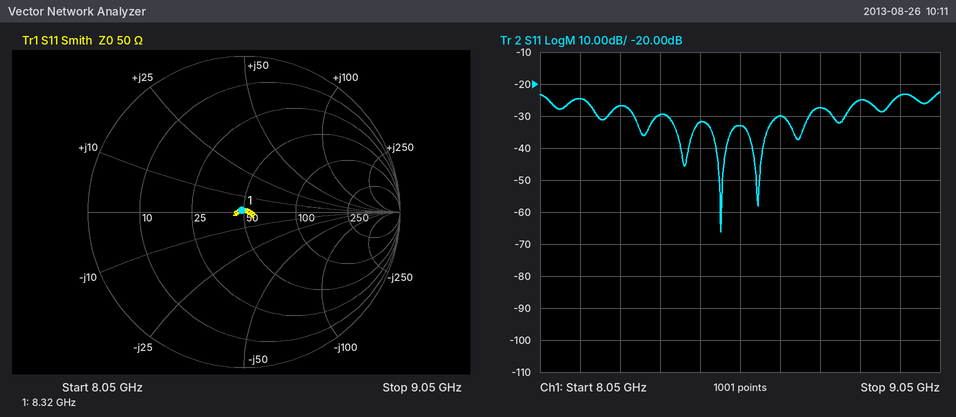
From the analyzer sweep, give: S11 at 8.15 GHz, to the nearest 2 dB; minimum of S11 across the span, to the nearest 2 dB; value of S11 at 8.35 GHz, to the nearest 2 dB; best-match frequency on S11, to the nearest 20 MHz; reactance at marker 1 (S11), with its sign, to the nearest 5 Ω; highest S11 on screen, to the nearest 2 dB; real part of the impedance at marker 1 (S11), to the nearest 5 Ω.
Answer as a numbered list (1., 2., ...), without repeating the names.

1. -24 dB
2. -66 dB
3. -30 dB
4. 8.50 GHz
5. 0 Ω
6. -22 dB
7. 50 Ω
